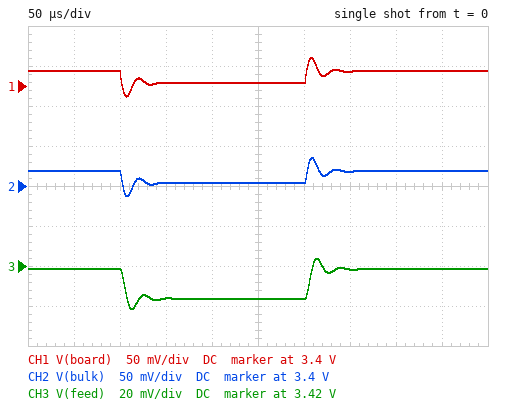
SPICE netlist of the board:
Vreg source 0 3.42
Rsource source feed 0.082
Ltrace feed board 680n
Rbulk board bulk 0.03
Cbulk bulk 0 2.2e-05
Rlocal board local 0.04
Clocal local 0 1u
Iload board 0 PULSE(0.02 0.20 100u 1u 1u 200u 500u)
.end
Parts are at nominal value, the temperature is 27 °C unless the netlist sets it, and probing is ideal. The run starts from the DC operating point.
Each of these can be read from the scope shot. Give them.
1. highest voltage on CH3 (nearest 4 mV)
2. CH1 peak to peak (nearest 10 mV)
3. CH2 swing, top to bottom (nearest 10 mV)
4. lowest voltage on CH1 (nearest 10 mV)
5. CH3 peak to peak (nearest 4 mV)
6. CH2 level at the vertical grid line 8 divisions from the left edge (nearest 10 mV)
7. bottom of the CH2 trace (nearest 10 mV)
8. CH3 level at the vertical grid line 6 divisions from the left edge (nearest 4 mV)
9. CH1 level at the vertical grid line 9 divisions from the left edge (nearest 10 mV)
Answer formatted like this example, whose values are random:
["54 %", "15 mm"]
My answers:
["3.424 V", "50 mV", "50 mV", "3.39 V", "24 mV", "3.42 V", "3.39 V", "3.404 V", "3.42 V"]
